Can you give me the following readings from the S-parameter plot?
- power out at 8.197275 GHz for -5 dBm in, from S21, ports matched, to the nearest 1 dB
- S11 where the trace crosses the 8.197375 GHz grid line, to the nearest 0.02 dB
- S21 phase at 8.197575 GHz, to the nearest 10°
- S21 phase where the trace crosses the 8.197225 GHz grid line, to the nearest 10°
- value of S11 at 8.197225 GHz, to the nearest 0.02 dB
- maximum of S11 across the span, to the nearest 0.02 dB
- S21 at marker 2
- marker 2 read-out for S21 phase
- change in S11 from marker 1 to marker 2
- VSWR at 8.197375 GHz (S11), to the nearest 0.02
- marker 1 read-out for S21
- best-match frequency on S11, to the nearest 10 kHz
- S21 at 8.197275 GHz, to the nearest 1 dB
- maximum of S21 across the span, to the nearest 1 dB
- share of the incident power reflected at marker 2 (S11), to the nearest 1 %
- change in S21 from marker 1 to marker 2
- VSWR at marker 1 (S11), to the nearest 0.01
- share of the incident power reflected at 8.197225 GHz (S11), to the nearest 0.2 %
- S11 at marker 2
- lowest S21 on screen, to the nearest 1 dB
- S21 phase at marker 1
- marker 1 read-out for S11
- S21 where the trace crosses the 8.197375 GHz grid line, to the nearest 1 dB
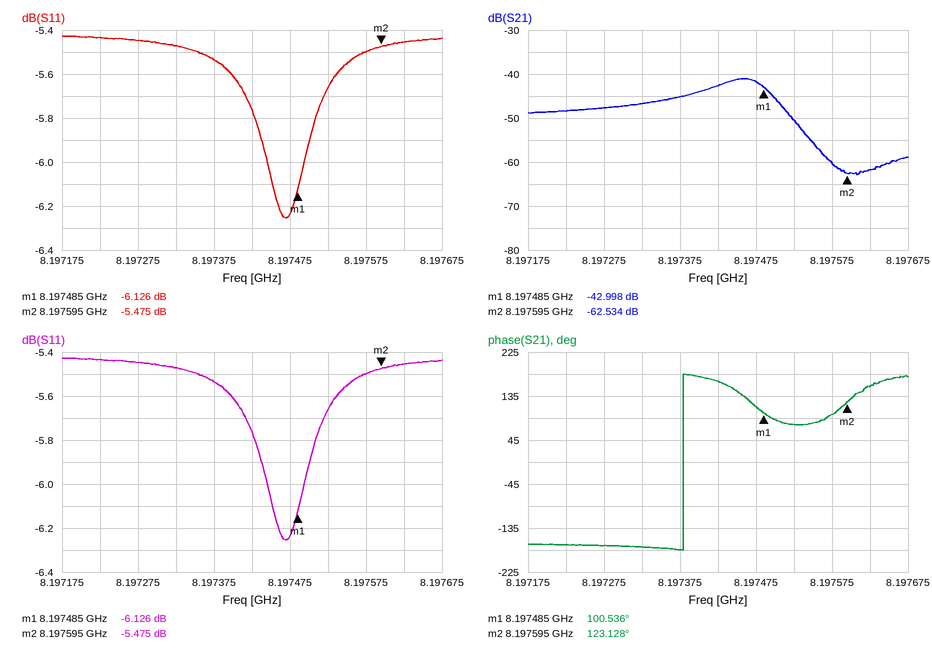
-53 dBm
-5.54 dB
100°
-170°
-5.44 dB
-5.42 dB
-62.534 dB
123.128°
0.651 dB
3.24
-42.998 dB
8.19747 GHz
-48 dB
-41 dB
28 %
-19.536 dB
2.95
28.6 %
-5.475 dB
-63 dB
100.536°
-6.126 dB
-45 dB
